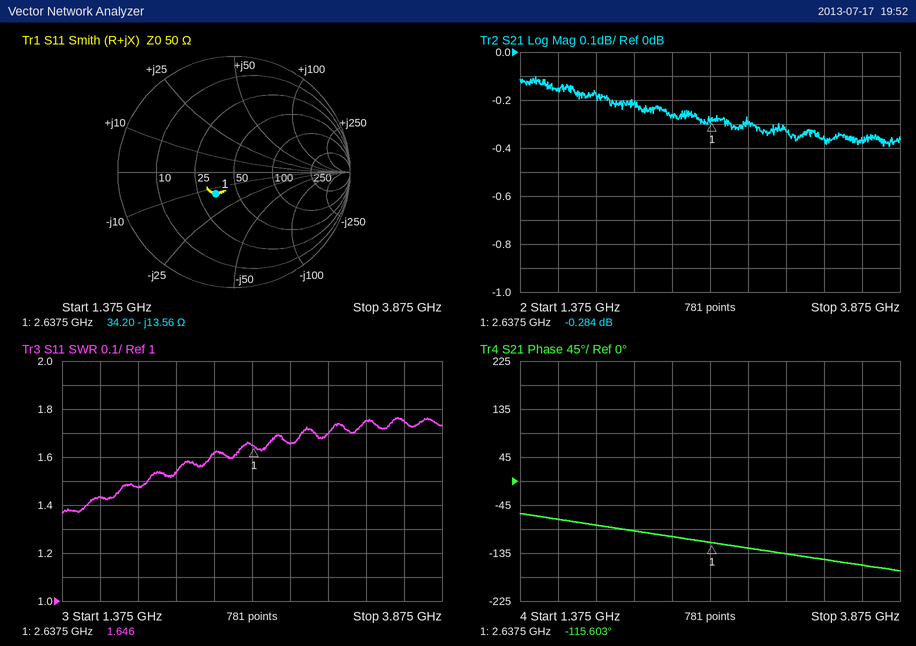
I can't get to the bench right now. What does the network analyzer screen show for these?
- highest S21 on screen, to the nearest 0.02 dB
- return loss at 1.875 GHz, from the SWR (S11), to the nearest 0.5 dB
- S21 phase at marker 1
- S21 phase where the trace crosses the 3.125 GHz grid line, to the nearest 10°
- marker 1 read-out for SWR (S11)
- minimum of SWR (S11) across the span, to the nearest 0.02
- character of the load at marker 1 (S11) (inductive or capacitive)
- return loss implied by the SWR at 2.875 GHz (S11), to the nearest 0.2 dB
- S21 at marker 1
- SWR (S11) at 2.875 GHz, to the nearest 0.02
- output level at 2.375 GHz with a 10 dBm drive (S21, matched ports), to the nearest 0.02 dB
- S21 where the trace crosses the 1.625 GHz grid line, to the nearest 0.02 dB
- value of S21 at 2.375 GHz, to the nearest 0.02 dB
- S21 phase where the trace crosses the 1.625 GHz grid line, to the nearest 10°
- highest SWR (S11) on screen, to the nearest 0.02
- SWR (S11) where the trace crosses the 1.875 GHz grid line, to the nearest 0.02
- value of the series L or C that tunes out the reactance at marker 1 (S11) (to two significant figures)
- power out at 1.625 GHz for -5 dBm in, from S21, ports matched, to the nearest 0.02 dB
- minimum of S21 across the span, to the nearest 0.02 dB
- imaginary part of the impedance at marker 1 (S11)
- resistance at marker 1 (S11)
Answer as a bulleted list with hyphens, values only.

- -0.10 dB
- 14.5 dB
- -115.603°
- -140°
- 1.646
- 1.36
- capacitive
- 12.2 dB
- -0.284 dB
- 1.66
- 9.74 dBm
- -0.16 dB
- -0.26 dB
- -70°
- 1.76
- 1.48
- 820 pH
- -5.16 dBm
- -0.40 dB
- -13.56 Ω
- 34.20 Ω
